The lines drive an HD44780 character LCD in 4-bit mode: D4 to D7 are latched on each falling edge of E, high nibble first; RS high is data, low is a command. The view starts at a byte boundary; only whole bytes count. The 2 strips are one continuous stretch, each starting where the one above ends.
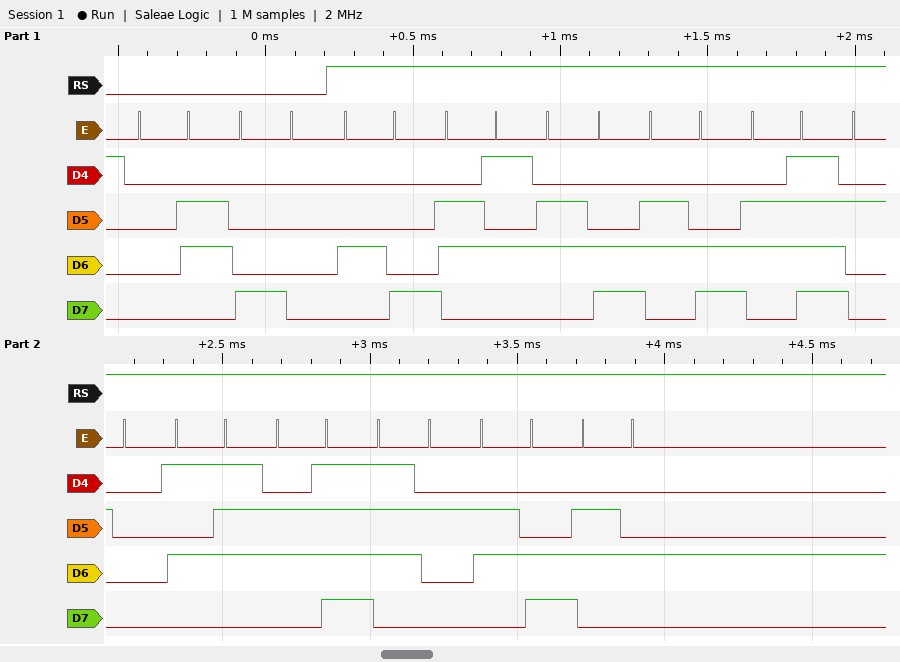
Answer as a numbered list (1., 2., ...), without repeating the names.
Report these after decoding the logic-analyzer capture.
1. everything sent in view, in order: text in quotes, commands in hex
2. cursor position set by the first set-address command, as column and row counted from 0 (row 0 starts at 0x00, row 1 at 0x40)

1. 0x06 0x80 "Hello World"
2. column 0, row 0
